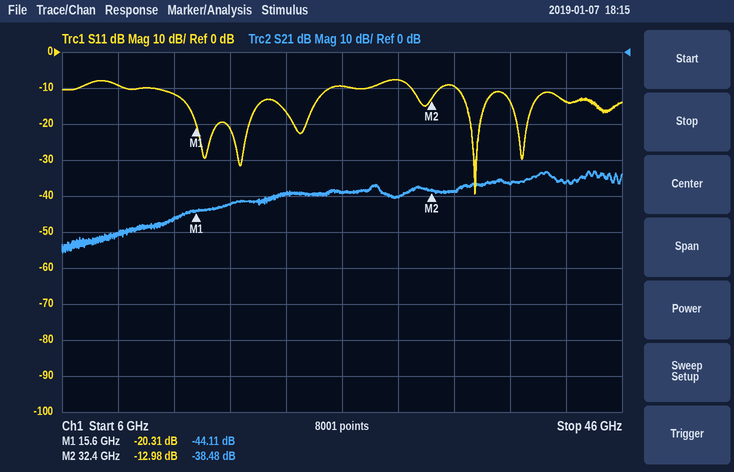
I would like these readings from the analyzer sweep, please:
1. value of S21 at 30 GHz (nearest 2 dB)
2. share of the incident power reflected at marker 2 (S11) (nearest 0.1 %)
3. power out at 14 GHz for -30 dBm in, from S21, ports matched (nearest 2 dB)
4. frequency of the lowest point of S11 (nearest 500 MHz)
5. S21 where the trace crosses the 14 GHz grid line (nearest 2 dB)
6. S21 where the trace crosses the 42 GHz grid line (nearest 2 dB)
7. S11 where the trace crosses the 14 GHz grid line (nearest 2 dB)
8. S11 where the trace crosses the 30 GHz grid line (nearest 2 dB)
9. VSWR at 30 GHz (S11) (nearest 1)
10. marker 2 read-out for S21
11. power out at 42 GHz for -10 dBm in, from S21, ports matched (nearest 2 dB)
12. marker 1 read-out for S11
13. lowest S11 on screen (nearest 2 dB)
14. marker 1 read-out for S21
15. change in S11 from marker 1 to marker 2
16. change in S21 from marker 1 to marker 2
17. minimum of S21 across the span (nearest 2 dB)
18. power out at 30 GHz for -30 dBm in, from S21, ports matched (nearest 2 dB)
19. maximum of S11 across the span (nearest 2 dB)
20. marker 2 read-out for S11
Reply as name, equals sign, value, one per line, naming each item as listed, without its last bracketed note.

value of S21 at 30 GHz = -40 dB
share of the incident power reflected at marker 2 (S11) = 5.0 %
power out at 14 GHz for -30 dBm in, from S21, ports matched = -76 dBm
frequency of the lowest point of S11 = 35.5 GHz
S21 where the trace crosses the 14 GHz grid line = -46 dB
S21 where the trace crosses the 42 GHz grid line = -36 dB
S11 where the trace crosses the 14 GHz grid line = -12 dB
S11 where the trace crosses the 30 GHz grid line = -8 dB
VSWR at 30 GHz (S11) = 2
marker 2 read-out for S21 = -38.48 dB
power out at 42 GHz for -10 dBm in, from S21, ports matched = -46 dBm
marker 1 read-out for S11 = -20.31 dB
lowest S11 on screen = -40 dB
marker 1 read-out for S21 = -44.11 dB
change in S11 from marker 1 to marker 2 = 7.33 dB
change in S21 from marker 1 to marker 2 = 5.63 dB
minimum of S21 across the span = -56 dB
power out at 30 GHz for -30 dBm in, from S21, ports matched = -70 dBm
maximum of S11 across the span = -8 dB
marker 2 read-out for S11 = -12.98 dB
